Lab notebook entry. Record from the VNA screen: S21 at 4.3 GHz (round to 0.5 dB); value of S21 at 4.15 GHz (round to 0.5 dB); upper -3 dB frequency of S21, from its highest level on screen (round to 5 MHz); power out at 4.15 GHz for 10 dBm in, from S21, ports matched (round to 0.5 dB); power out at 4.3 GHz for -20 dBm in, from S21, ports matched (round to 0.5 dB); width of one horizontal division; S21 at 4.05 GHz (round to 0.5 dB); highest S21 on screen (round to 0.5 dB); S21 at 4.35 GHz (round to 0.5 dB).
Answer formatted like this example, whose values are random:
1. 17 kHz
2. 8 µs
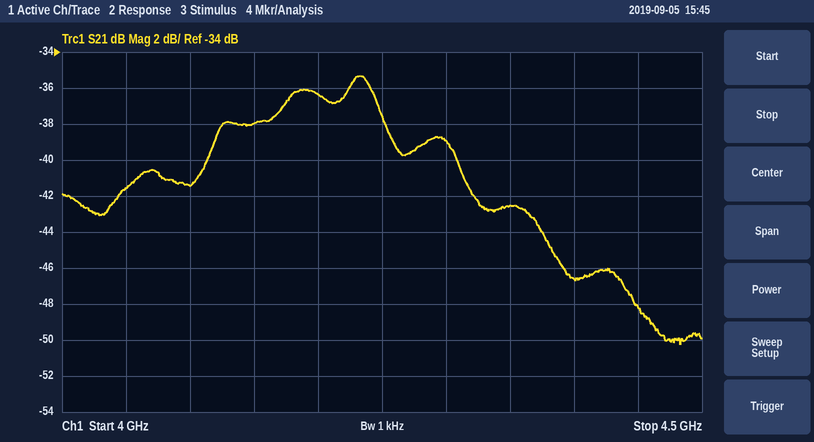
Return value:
1. -39.0 dB
2. -38.0 dB
3. 4.255 GHz
4. -28.0 dBm
5. -59.0 dBm
6. 50 MHz
7. -41.5 dB
8. -35.5 dB
9. -42.5 dB
